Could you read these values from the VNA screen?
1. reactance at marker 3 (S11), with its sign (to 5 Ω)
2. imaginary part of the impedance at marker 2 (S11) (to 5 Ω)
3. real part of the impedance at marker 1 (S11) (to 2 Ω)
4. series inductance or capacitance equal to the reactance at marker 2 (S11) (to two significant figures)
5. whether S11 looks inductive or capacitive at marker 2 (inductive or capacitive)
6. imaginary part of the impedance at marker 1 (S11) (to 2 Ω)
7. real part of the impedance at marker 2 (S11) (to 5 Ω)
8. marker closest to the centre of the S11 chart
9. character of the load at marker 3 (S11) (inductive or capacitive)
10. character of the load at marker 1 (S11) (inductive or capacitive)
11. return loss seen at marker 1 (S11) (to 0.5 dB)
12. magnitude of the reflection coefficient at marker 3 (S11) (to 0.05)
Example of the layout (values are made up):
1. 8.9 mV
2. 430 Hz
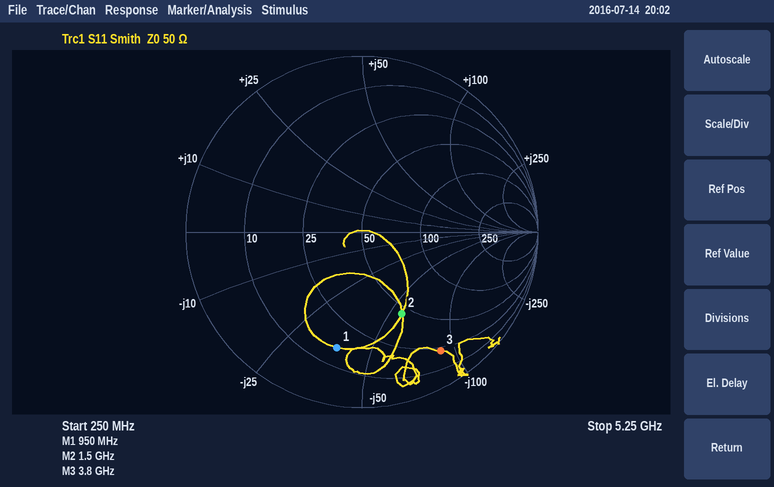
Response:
1. -90 Ω
2. -55 Ω
3. 16 Ω
4. 1.9 pF
5. capacitive
6. -38 Ω
7. 45 Ω
8. marker 2
9. capacitive
10. capacitive
11. 3.5 dB
12. 0.80
